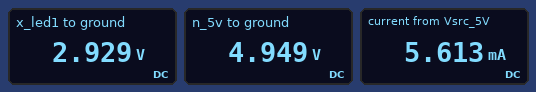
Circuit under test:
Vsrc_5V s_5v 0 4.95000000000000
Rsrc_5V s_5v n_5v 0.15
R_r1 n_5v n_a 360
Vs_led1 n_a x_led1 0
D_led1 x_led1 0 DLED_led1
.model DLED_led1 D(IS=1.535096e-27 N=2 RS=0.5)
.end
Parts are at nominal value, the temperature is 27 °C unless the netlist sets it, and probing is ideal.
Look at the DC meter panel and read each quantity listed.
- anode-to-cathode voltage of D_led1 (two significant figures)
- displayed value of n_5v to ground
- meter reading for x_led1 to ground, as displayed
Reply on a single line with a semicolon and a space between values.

2.9 V; 4.949 V; 2.929 V
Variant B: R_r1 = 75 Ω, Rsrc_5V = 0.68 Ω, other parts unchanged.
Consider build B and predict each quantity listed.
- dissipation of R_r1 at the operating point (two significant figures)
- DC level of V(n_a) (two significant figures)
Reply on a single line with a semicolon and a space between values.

49 mW; 3.0 V
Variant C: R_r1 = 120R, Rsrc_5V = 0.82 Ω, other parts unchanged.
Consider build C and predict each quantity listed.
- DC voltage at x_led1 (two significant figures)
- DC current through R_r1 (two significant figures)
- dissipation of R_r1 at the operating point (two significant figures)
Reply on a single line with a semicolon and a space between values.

3.0 V; 16 mA; 32 mW
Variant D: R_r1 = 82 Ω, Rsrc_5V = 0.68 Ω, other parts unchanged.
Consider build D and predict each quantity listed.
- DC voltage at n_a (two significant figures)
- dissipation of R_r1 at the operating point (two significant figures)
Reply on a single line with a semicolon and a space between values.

3.0 V; 45 mW
